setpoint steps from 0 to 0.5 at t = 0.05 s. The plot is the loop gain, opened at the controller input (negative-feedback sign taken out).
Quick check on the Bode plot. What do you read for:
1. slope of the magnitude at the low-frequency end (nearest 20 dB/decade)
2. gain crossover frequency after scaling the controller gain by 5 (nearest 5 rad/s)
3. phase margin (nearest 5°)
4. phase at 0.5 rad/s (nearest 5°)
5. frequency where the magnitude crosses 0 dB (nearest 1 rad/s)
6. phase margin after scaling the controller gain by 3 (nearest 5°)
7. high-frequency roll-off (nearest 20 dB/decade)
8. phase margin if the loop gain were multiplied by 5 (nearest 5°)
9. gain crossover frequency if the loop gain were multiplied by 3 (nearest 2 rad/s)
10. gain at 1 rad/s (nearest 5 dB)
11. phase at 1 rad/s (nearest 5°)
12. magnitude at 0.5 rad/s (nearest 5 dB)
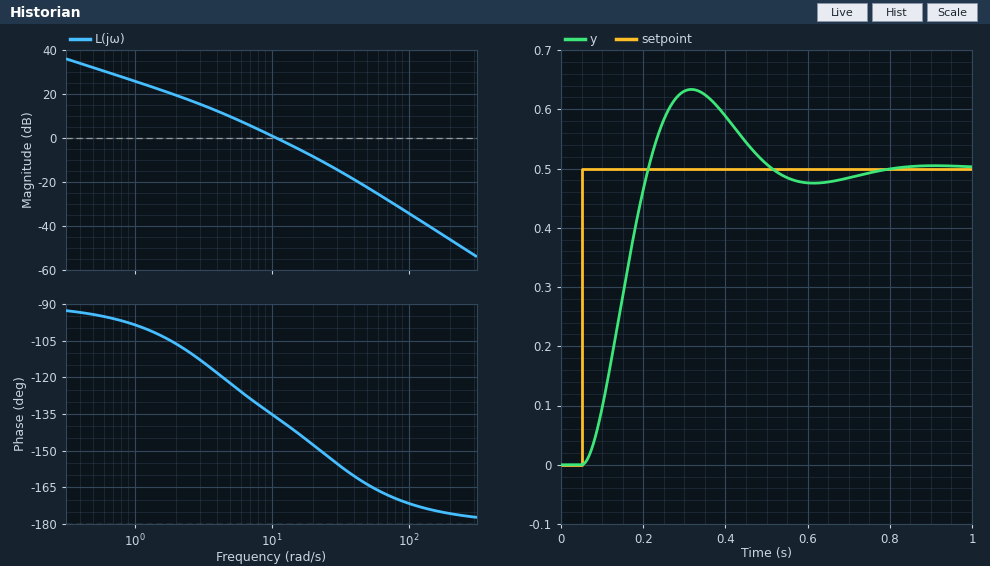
-20 dB/decade
30 rad/s
45°
-95°
11 rad/s
30°
-40 dB/decade
25°
22 rad/s
25 dB
-100°
30 dB
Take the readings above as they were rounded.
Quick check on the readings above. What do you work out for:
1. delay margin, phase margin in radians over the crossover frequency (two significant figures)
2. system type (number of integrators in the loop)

0.071 s
1
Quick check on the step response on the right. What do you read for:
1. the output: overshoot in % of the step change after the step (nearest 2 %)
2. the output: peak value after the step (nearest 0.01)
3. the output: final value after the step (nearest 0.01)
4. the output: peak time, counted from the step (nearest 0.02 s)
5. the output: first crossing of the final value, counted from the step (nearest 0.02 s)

26 %
0.63
0.50
0.26 s
0.16 s
